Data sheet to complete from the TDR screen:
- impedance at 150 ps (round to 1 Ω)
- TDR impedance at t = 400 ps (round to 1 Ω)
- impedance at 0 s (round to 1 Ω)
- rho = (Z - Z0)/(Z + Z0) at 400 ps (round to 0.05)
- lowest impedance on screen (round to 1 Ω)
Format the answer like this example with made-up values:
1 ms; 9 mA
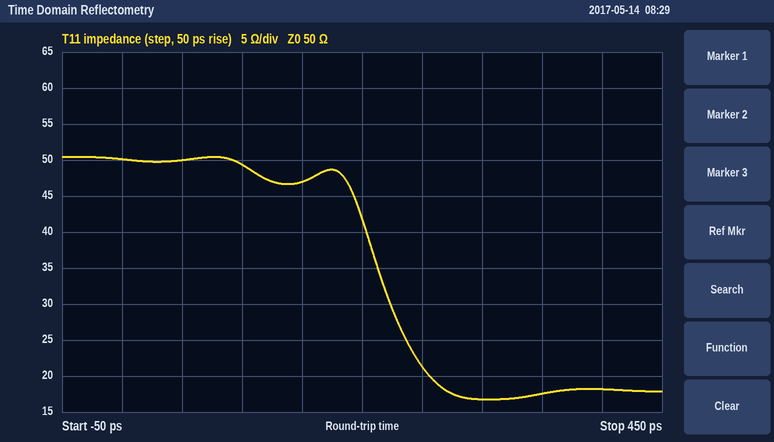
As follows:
47 Ω; 18 Ω; 50 Ω; -0.45; 17 Ω
